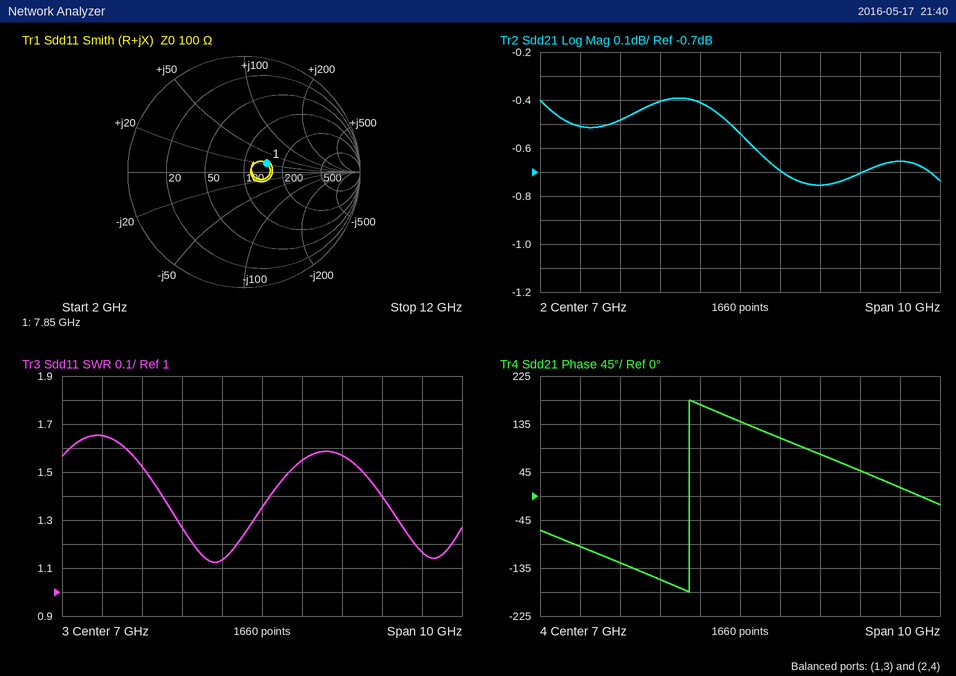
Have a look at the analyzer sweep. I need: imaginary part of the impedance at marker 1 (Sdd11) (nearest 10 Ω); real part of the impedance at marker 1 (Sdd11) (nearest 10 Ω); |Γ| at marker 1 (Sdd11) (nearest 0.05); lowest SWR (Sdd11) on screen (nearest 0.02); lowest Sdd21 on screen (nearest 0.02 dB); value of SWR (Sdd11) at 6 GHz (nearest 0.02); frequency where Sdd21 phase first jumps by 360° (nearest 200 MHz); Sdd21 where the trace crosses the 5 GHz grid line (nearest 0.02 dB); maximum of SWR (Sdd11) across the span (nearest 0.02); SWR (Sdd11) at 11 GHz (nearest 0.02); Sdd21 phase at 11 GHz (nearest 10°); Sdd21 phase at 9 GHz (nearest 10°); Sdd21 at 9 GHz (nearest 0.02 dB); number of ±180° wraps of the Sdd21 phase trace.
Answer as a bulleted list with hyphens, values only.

- +20 Ω
- 150 Ω
- 0.20
- 1.12
- -0.76 dB
- 1.14
- 5.8 GHz
- -0.40 dB
- 1.66
- 1.16
- 20°
- 80°
- -0.76 dB
- 1
